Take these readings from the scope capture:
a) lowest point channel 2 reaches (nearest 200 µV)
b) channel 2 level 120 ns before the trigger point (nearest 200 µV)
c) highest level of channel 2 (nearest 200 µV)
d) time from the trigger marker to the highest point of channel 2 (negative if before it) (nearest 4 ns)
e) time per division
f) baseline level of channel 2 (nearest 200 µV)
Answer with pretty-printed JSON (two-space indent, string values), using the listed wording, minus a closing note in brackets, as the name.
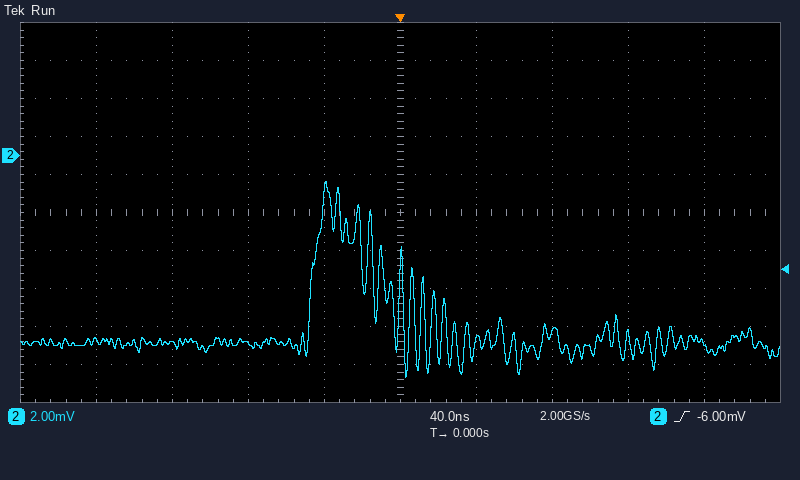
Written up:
{
  "lowest point channel 2 reaches": "-11.6 mV",
  "channel 2 level 120 ns before the trigger point": "-10.0 mV",
  "highest level of channel 2": "-1.4 mV",
  "time from the trigger marker to the highest point of channel 2 (negative if before it)": "-40 ns",
  "time per division": "40 ns",
  "baseline level of channel 2": "-9.8 mV"
}
